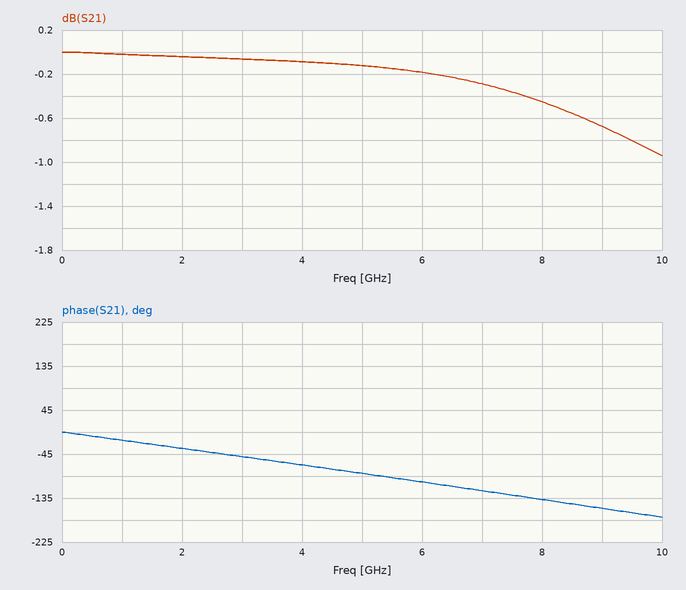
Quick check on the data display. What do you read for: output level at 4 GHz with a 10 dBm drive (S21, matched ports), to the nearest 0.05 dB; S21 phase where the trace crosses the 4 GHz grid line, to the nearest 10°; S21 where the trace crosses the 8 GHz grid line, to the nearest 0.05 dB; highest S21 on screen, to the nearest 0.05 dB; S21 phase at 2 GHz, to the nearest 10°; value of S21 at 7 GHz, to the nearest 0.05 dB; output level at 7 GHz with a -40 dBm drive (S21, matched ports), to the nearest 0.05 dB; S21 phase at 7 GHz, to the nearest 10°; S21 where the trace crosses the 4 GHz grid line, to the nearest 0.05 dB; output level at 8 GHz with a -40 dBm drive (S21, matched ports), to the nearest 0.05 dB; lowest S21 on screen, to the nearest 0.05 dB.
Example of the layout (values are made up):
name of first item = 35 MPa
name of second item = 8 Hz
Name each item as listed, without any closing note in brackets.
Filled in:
output level at 4 GHz with a 10 dBm drive (S21, matched ports), to the nearest 0.05 dB = 9.90 dBm
S21 phase where the trace crosses the 4 GHz grid line, to the nearest 10° = -70°
S21 where the trace crosses the 8 GHz grid line, to the nearest 0.05 dB = -0.45 dB
highest S21 on screen, to the nearest 0.05 dB = 0.00 dB
S21 phase at 2 GHz, to the nearest 10° = -30°
value of S21 at 7 GHz, to the nearest 0.05 dB = -0.30 dB
output level at 7 GHz with a -40 dBm drive (S21, matched ports), to the nearest 0.05 dB = -40.30 dBm
S21 phase at 7 GHz, to the nearest 10° = -120°
S21 where the trace crosses the 4 GHz grid line, to the nearest 0.05 dB = -0.10 dB
output level at 8 GHz with a -40 dBm drive (S21, matched ports), to the nearest 0.05 dB = -40.45 dBm
lowest S21 on screen, to the nearest 0.05 dB = -0.95 dB
